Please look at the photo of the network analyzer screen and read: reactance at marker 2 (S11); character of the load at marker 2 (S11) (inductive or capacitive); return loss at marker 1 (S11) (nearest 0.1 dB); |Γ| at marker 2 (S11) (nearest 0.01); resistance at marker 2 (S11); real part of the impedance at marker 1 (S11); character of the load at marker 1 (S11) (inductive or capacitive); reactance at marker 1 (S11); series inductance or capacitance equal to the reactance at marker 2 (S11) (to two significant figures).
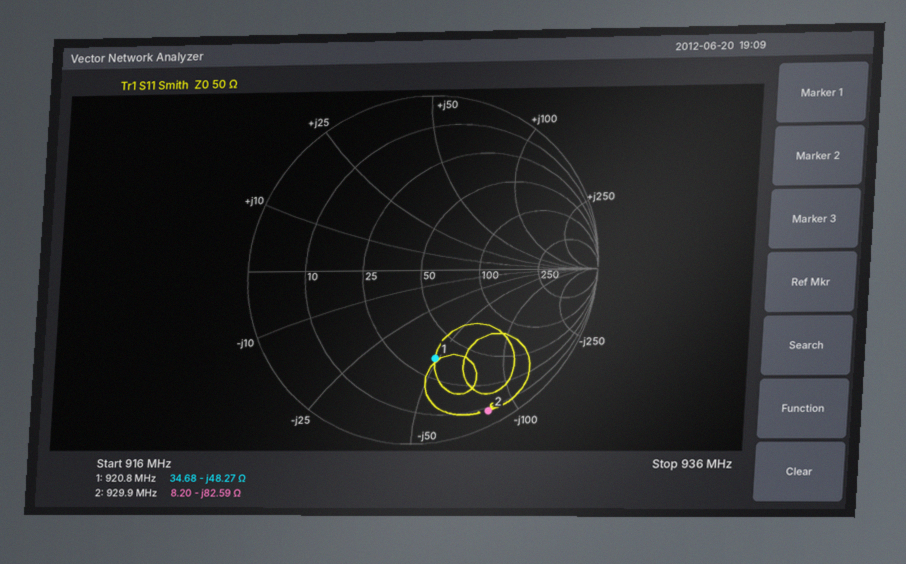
-82.59 Ω
capacitive
5.7 dB
0.92
8.20 Ω
34.68 Ω
capacitive
-48.27 Ω
2.1 pF
